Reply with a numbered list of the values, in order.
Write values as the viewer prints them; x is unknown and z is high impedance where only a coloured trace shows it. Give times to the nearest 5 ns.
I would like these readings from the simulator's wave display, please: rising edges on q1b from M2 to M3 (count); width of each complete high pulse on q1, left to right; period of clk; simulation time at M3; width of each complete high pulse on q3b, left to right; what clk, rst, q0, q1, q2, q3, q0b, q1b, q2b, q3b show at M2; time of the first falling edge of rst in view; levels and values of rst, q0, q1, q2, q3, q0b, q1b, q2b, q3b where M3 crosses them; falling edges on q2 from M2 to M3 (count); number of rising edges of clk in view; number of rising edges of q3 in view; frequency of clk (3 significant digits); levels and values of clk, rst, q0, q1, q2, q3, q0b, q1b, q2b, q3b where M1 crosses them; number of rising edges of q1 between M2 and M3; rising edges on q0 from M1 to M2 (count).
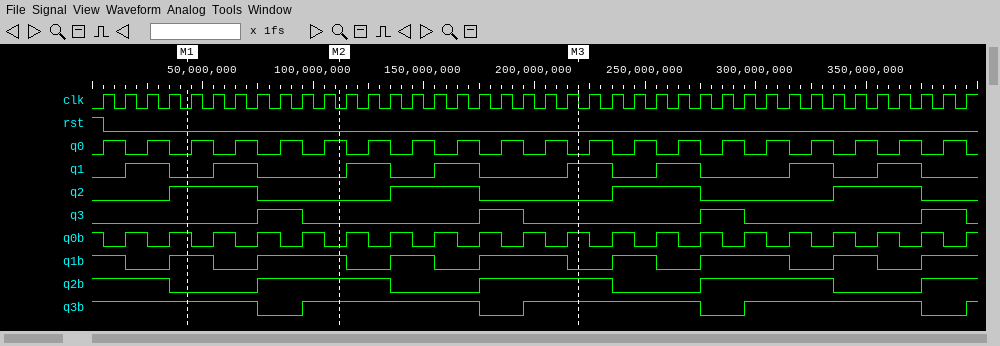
1. 2
2. 20 ns, 20 ns, 20 ns, 20 ns, 20 ns, 20 ns, 20 ns, 20 ns
3. 10 ns
4. 220 ns
5. 80 ns, 80 ns, 80 ns
6. clk=0, rst=0, q0=1, q1=0, q2=0, q3=0, q0b=0, q1b=1, q2b=1, q3b=1
7. 5 ns
8. rst=0, q0=0, q1=1, q2=0, q3=0, q0b=1, q1b=0, q2b=1, q3b=1
9. 1
10. 40
11. 4
12. 100 MHz
13. clk=0, rst=0, q0=0, q1=0, q2=1, q3=0, q0b=1, q1b=1, q2b=0, q3b=1
14. 3
15. 4
